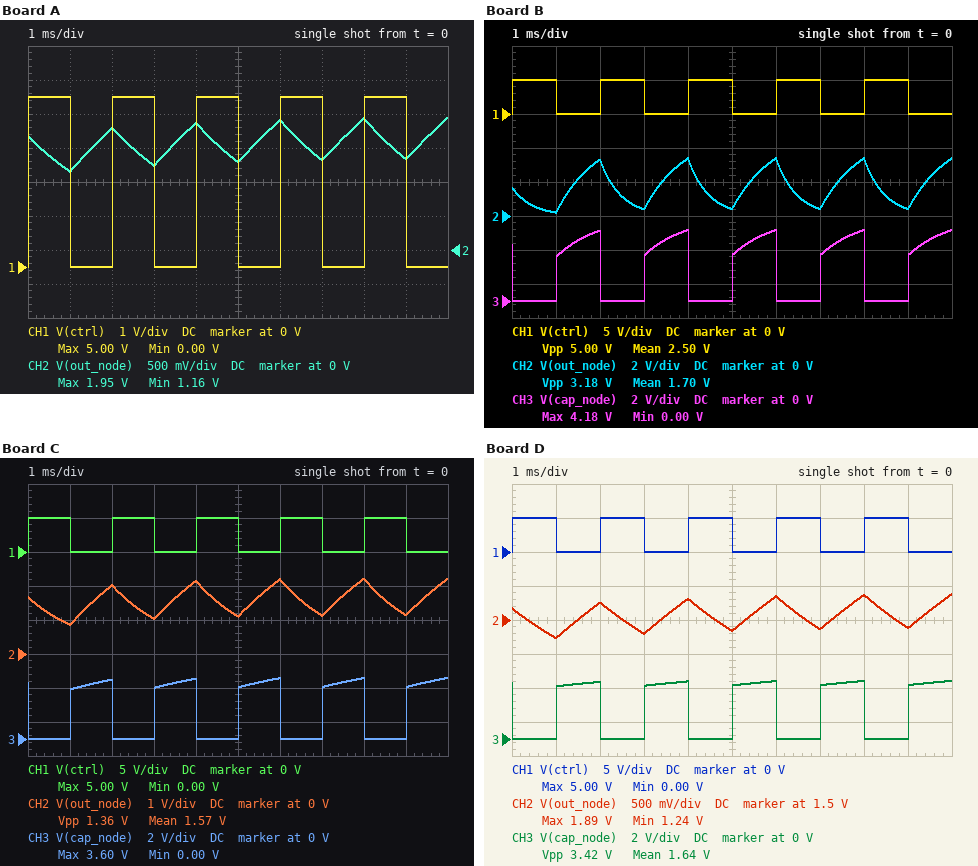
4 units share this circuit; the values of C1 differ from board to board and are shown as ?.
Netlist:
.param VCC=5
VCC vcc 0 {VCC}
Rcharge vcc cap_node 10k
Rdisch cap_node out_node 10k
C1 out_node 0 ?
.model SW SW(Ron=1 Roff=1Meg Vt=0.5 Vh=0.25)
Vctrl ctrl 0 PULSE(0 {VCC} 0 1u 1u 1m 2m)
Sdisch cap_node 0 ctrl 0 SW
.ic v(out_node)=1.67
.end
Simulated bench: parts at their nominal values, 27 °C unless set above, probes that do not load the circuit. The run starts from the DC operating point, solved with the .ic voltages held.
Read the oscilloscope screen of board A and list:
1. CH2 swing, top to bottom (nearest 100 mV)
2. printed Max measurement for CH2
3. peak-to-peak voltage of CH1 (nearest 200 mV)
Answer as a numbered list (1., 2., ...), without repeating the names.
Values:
1. 800 mV
2. 1.95 V
3. 5.0 V
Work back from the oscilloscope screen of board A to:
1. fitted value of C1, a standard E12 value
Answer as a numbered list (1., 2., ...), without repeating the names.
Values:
1. 270 nF
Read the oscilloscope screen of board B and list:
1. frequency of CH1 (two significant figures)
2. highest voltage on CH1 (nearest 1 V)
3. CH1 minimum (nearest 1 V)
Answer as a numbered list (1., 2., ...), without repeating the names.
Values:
1. 500 Hz
2. 5 V
3. 0 V
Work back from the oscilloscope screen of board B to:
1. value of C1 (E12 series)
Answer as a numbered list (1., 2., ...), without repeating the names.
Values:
1. 47 nF
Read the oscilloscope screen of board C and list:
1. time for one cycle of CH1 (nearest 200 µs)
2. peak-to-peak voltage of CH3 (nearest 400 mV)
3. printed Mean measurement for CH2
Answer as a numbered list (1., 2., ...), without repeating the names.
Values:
1. 2.0 ms
2. 3.6 V
3. 1.57 V
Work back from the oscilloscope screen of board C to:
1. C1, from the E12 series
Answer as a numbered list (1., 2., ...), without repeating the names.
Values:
1. 150 nF
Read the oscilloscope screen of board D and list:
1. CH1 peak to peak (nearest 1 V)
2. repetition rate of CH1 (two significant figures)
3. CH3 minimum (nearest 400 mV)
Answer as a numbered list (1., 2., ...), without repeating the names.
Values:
1. 5 V
2. 500 Hz
3. 0 V
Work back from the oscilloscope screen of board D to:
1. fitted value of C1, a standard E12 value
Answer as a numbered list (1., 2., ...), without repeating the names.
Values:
1. 330 nF
